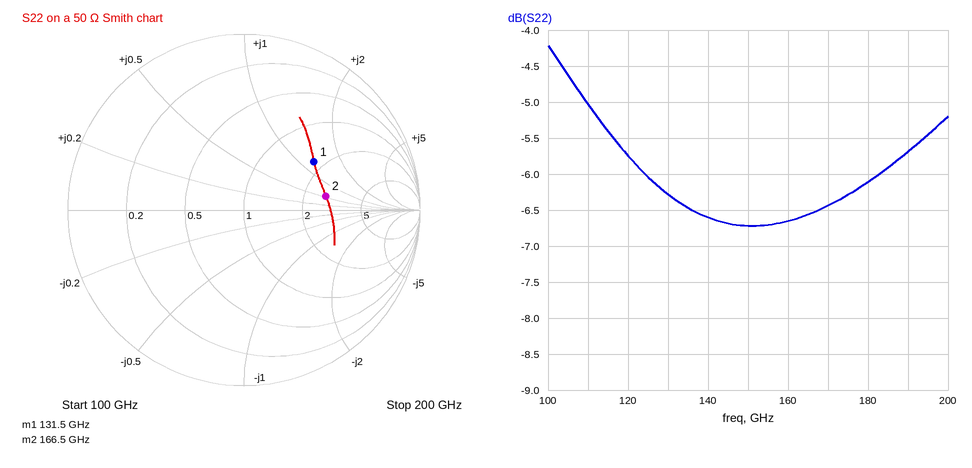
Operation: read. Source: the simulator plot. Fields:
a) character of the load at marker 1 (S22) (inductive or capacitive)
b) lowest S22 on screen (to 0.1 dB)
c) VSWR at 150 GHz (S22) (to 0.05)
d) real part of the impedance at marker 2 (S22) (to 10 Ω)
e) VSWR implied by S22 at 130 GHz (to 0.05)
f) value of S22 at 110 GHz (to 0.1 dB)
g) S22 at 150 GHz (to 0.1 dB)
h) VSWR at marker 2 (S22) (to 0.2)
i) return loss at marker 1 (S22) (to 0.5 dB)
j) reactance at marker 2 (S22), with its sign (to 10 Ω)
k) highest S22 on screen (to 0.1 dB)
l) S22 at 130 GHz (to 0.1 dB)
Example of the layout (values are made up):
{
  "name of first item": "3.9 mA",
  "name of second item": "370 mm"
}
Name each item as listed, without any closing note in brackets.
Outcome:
{
  "character of the load at marker 1 (S22)": "inductive",
  "lowest S22 on screen": "-6.7 dB",
  "VSWR at 150 GHz (S22)": "2.70",
  "real part of the impedance at marker 2 (S22)": "130 Ω",
  "VSWR implied by S22 at 130 GHz": "2.90",
  "value of S22 at 110 GHz": "-5.0 dB",
  "S22 at 150 GHz": "-6.7 dB",
  "VSWR at marker 2 (S22)": "2.8",
  "return loss at marker 1 (S22)": "6.5 dB",
  "reactance at marker 2 (S22), with its sign": "+30 Ω",
  "highest S22 on screen": "-4.2 dB",
  "S22 at 130 GHz": "-6.3 dB"
}
